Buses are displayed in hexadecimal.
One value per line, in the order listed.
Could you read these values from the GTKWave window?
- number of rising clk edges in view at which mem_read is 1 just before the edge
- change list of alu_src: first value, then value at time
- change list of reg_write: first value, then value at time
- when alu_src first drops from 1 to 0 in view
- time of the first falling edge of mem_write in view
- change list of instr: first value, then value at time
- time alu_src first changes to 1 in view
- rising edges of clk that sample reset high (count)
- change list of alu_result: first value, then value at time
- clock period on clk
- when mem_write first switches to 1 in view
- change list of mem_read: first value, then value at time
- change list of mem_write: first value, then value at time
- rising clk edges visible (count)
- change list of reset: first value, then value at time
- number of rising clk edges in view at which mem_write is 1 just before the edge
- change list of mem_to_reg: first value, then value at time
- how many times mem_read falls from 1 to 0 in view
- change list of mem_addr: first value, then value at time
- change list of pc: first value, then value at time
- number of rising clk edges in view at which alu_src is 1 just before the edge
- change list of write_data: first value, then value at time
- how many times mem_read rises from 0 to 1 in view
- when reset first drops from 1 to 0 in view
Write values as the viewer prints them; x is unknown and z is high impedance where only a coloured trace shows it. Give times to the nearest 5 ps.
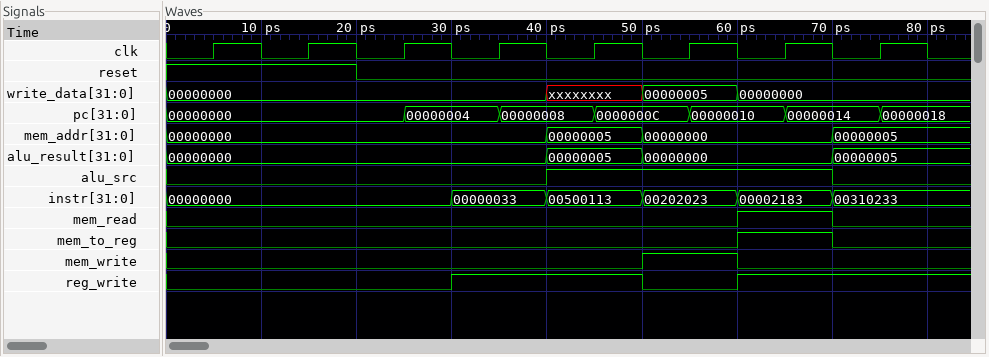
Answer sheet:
1
0, 1 at 40 ps, 0 at 70 ps
0, 1 at 30 ps, 0 at 50 ps, 1 at 60 ps
70 ps
60 ps
00000000, 00000033 at 30 ps, 00500113 at 40 ps, 00202023 at 50 ps, 00002183 at 60 ps, 00310233 at 70 ps
40 ps
2
00000000, 00000005 at 40 ps, 00000000 at 50 ps, 00000005 at 70 ps
10 ps
50 ps
0, 1 at 60 ps, 0 at 70 ps
0, 1 at 50 ps, 0 at 60 ps
8
1, 0 at 20 ps
1
0, 1 at 60 ps, 0 at 70 ps
1
00000000, 00000005 at 40 ps, 00000000 at 50 ps, 00000005 at 70 ps
00000000, 00000004 at 25 ps, 00000008 at 35 ps, 0000000C at 45 ps, 00000010 at 55 ps, 00000014 at 65 ps, 00000018 at 75 ps
3
00000000, xxxxxxxx at 40 ps, 00000005 at 50 ps, 00000000 at 60 ps
1
20 ps
